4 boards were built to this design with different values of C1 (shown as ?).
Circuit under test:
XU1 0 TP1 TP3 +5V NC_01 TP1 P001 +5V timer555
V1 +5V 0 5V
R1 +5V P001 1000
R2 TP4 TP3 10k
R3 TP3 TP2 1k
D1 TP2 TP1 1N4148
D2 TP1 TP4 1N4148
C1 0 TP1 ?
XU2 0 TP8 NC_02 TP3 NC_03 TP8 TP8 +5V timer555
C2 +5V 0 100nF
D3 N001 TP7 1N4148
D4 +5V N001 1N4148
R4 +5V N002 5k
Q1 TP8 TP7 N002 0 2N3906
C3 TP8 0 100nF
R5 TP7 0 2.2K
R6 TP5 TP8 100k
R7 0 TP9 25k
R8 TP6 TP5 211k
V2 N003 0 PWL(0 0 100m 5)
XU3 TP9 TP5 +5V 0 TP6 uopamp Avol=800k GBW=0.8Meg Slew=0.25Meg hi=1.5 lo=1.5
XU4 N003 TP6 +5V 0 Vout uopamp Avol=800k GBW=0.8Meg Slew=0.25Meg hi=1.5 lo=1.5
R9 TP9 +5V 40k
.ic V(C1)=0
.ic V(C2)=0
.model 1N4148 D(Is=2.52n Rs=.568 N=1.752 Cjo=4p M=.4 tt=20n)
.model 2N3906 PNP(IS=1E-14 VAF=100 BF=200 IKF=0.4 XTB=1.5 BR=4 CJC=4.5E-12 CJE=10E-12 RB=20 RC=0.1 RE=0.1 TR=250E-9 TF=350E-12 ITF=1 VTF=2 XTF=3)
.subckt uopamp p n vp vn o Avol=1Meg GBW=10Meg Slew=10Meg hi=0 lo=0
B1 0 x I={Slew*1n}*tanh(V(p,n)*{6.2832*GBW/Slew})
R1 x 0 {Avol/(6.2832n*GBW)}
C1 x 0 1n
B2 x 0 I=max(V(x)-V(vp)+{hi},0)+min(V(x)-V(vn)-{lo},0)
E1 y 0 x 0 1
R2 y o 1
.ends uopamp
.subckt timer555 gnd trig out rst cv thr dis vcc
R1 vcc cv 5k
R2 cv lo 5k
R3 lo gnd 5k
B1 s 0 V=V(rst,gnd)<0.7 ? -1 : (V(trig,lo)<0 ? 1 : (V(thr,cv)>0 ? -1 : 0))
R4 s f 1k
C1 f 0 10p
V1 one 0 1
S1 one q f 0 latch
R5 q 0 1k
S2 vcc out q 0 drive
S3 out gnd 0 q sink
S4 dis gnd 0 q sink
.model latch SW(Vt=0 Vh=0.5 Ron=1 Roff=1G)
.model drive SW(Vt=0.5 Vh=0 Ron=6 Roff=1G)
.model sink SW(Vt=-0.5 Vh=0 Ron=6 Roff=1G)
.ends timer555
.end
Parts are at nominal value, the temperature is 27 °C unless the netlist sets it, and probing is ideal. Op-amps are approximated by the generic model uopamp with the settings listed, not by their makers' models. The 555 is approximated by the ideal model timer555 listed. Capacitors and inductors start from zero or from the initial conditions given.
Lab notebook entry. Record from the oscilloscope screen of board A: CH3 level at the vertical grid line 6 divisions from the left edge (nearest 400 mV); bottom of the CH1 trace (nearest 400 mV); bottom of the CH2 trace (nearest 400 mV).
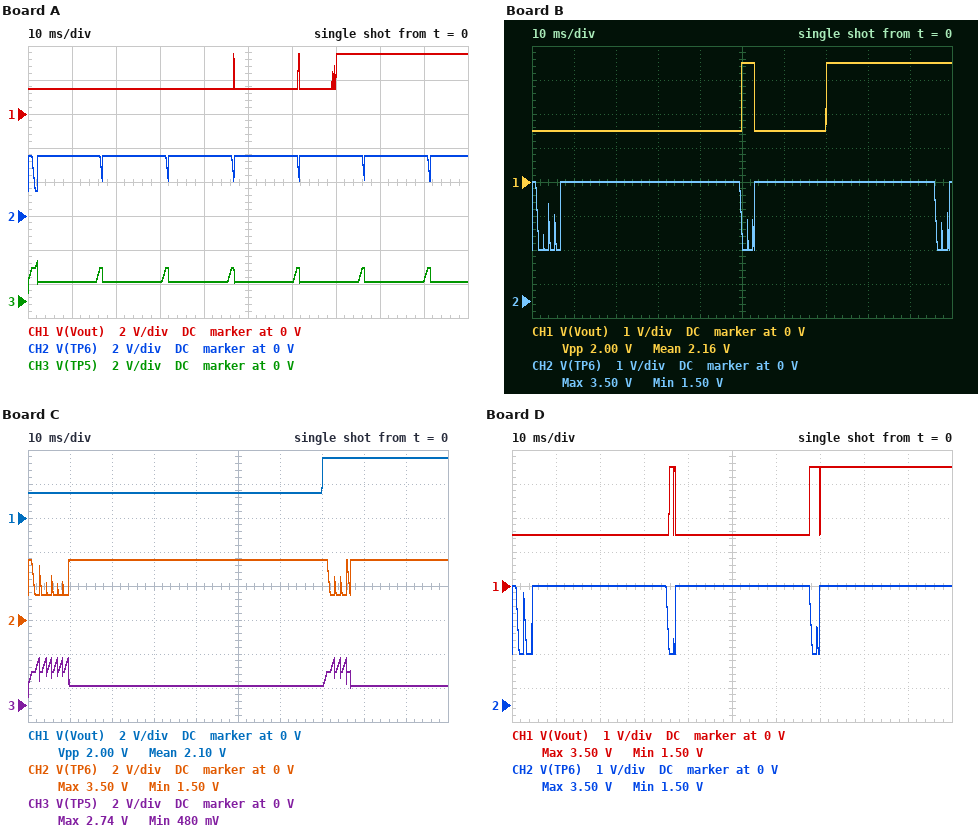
1.2 V
1.6 V
1.6 V
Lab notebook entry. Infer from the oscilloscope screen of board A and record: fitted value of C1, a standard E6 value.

1.5 µF
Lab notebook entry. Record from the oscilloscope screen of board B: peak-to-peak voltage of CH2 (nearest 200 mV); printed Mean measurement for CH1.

2.0 V
2.16 V
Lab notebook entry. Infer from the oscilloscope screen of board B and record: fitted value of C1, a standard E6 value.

4.7 µF
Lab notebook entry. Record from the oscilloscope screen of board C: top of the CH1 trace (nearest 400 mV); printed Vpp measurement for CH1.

3.6 V
2.00 V
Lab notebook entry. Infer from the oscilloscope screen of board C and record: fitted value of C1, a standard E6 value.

6.8 µF
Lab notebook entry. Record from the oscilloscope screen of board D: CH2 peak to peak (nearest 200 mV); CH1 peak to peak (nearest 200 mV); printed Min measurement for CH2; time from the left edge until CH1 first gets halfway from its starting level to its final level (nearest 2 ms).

2.0 V
2.0 V
1.50 V
36 ms
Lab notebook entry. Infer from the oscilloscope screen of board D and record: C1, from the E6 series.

3.3 µF
